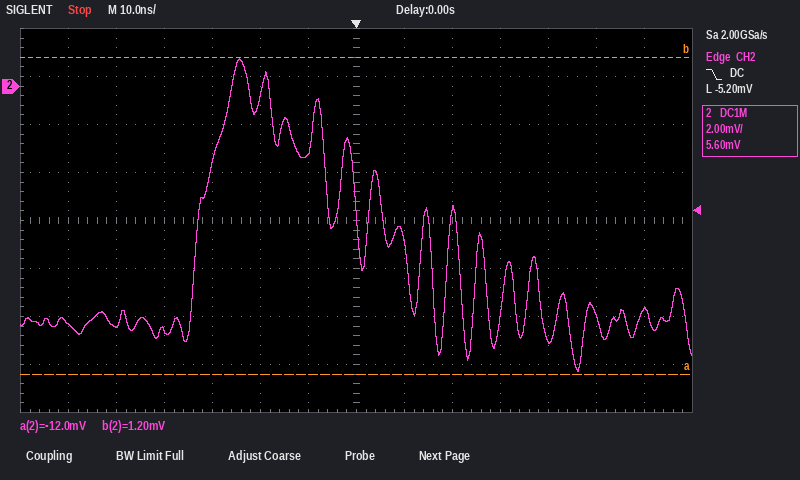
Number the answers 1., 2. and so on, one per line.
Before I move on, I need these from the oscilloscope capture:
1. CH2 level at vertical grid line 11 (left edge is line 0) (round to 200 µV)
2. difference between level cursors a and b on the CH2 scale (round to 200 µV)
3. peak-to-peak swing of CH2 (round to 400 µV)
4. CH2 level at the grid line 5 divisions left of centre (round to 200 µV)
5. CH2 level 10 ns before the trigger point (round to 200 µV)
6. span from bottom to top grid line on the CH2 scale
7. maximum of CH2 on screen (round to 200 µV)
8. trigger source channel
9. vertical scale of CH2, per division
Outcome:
1. -10.6 mV
2. 13.2 mV
3. 13.2 mV
4. -10.0 mV
5. -2.8 mV
6. 16 mV
7. 1.2 mV
8. CH2
9. 2 mV
